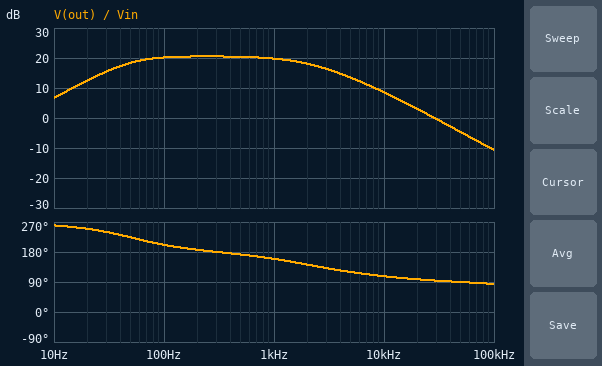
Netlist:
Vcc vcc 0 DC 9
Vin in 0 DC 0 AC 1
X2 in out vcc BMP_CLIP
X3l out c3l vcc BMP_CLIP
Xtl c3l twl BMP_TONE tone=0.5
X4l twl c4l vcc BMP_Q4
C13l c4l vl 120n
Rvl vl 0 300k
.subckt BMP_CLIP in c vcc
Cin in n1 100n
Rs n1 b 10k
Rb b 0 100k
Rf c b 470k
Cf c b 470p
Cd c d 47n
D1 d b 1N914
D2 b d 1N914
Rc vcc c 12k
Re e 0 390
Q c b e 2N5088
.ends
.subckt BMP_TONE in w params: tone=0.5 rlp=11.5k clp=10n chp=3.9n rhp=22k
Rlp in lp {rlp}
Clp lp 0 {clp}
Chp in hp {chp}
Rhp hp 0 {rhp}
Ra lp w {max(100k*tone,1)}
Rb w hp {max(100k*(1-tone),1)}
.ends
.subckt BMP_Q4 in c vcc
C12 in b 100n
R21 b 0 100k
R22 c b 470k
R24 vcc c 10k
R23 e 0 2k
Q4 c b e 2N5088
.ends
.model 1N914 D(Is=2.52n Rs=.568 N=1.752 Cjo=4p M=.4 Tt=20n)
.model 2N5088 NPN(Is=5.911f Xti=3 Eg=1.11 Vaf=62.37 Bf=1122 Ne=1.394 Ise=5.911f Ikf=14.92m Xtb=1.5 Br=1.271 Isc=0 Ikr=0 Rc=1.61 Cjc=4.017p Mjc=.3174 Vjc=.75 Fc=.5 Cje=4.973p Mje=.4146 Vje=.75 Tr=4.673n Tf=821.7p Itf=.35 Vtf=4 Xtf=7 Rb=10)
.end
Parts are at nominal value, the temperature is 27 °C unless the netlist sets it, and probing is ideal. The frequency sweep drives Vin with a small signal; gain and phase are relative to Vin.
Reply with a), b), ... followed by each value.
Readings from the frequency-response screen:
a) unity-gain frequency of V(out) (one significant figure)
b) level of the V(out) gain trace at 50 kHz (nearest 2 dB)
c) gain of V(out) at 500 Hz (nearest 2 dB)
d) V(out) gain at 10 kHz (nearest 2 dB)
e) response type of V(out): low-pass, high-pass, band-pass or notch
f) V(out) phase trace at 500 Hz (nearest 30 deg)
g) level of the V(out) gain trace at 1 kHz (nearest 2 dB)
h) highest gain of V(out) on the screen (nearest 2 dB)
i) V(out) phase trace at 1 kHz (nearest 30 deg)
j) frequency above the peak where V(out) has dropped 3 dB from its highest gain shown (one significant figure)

a) 30 kHz
b) -4 dB
c) 20 dB
d) 8 dB
e) band-pass
f) 180 deg
g) 20 dB
h) 20 dB
i) 150 deg
j) 2 kHz
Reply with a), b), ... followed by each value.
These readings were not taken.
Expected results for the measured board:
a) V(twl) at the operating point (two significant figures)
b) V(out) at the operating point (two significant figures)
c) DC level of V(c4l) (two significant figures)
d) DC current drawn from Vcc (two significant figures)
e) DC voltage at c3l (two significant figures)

a) 2.5 V
b) 4.7 V
c) 6.5 V
d) 970 µA
e) 4.6 V
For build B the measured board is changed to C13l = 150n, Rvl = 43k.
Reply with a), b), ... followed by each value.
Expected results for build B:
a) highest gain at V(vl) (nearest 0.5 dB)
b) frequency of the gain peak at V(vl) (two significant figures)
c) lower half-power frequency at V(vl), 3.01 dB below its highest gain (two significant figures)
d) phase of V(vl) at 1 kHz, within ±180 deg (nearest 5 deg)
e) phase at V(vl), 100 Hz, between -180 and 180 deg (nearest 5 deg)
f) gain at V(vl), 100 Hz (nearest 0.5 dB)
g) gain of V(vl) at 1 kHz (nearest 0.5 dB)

a) 43.5 dB
b) 230 Hz
c) 73 Hz
d) 125 deg
e) -110 deg
f) 42.0 dB
g) 39.0 dB
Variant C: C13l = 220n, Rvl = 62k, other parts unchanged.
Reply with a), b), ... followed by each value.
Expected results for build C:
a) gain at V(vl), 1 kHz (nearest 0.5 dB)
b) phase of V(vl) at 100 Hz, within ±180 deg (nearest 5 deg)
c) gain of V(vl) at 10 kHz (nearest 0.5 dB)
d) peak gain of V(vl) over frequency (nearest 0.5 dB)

a) 39.5 dB
b) -115 deg
c) 18.5 dB
d) 44.0 dB
